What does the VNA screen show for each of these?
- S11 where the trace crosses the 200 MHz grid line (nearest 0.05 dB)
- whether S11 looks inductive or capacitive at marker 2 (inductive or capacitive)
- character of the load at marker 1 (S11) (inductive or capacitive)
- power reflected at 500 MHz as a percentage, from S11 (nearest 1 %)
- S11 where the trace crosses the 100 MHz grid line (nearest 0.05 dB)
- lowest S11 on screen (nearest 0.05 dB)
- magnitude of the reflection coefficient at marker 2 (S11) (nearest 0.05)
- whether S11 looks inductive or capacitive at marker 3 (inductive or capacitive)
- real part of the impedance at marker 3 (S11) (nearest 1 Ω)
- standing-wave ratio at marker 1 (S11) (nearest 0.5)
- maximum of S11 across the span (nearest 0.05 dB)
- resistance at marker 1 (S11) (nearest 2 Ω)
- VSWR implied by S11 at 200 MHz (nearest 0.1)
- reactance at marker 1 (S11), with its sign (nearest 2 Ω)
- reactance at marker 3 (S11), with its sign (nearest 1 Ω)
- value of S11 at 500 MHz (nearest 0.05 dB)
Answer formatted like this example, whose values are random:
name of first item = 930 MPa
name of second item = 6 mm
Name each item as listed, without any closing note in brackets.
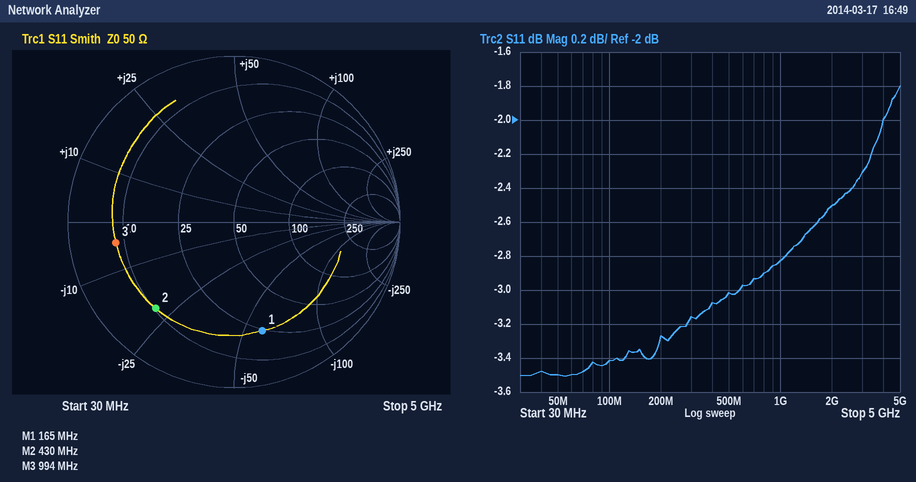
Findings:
S11 where the trace crosses the 200 MHz grid line = -3.25 dB
whether S11 looks inductive or capacitive at marker 2 = capacitive
character of the load at marker 1 (S11) = capacitive
power reflected at 500 MHz as a percentage, from S11 = 50 %
S11 where the trace crosses the 100 MHz grid line = -3.40 dB
lowest S11 on screen = -3.50 dB
magnitude of the reflection coefficient at marker 2 (S11) = 0.70
whether S11 looks inductive or capacitive at marker 3 = capacitive
real part of the impedance at marker 3 (S11) = 8 Ω
standing-wave ratio at marker 1 (S11) = 5.0
maximum of S11 across the span = -1.80 dB
resistance at marker 1 (S11) = 24 Ω
VSWR implied by S11 at 200 MHz = 5.4
reactance at marker 1 (S11), with its sign = -58 Ω
reactance at marker 3 (S11), with its sign = -4 Ω
value of S11 at 500 MHz = -3.00 dB
